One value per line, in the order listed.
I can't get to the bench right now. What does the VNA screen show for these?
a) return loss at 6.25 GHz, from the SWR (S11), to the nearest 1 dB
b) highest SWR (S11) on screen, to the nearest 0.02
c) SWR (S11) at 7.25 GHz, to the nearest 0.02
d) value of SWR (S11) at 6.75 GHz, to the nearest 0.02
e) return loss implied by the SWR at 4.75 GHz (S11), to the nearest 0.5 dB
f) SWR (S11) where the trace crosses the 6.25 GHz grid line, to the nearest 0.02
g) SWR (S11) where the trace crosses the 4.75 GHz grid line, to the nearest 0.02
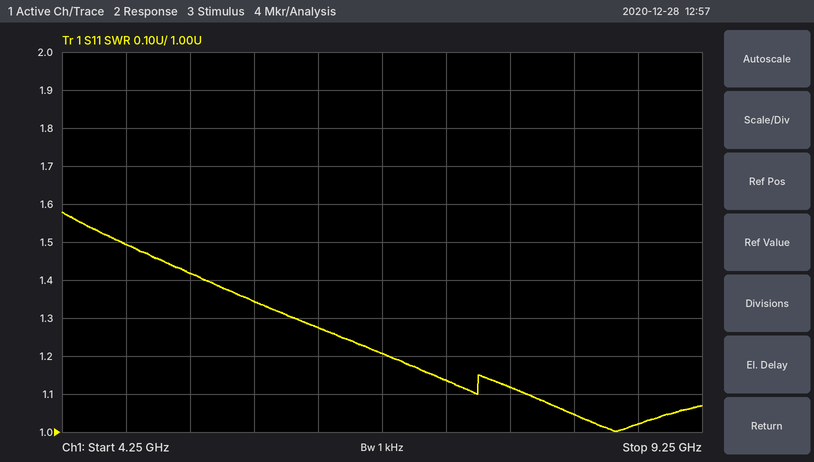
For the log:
18 dB
1.58
1.14
1.20
14.0 dB
1.28
1.50
